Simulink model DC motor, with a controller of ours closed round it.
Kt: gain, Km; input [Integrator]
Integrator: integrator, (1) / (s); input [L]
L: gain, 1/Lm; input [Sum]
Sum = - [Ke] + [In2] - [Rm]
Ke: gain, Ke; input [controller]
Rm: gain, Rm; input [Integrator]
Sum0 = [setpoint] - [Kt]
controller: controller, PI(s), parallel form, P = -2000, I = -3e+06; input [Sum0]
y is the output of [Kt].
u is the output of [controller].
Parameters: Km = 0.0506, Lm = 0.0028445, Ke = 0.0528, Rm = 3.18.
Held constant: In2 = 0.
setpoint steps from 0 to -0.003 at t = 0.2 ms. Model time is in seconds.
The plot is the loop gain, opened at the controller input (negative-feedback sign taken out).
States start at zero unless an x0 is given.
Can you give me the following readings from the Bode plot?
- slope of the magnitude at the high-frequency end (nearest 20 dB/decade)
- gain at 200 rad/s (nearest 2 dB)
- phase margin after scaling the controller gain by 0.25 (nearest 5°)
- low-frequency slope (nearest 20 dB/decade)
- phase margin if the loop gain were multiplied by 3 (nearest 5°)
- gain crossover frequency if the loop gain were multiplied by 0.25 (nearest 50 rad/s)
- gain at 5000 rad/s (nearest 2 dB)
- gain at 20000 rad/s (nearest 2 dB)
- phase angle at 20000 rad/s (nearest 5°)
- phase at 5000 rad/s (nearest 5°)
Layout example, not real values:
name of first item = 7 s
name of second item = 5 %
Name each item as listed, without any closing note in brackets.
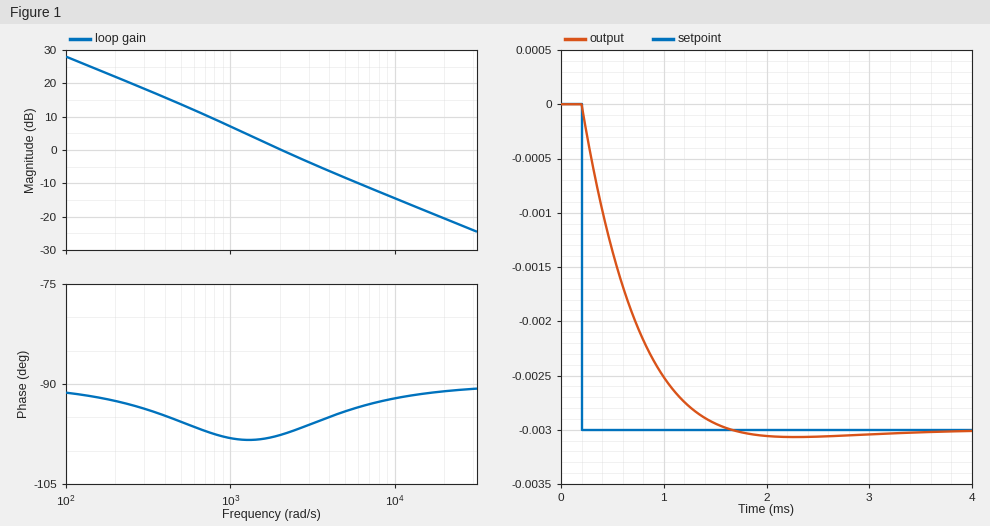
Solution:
slope of the magnitude at the high-frequency end = -20 dB/decade
gain at 200 rad/s = 22 dB
phase margin after scaling the controller gain by 0.25 = 85°
low-frequency slope = -20 dB/decade
phase margin if the loop gain were multiplied by 3 = 85°
gain crossover frequency if the loop gain were multiplied by 0.25 = 600 rad/s
gain at 5000 rad/s = -8 dB
gain at 20000 rad/s = -20 dB
phase angle at 20000 rad/s = -90°
phase at 5000 rad/s = -95°
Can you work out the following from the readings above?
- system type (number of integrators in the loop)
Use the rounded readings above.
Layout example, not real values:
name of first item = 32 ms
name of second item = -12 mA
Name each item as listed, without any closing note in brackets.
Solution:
system type = 1
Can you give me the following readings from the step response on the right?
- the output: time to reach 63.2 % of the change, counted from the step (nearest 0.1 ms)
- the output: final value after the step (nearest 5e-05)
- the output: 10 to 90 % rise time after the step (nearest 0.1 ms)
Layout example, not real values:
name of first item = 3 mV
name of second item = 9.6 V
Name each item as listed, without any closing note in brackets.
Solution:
the output: time to reach 63.2 % of the change, counted from the step = 0.5 ms
the output: final value after the step = -0.00300
the output: 10 to 90 % rise time after the step = 0.9 ms
